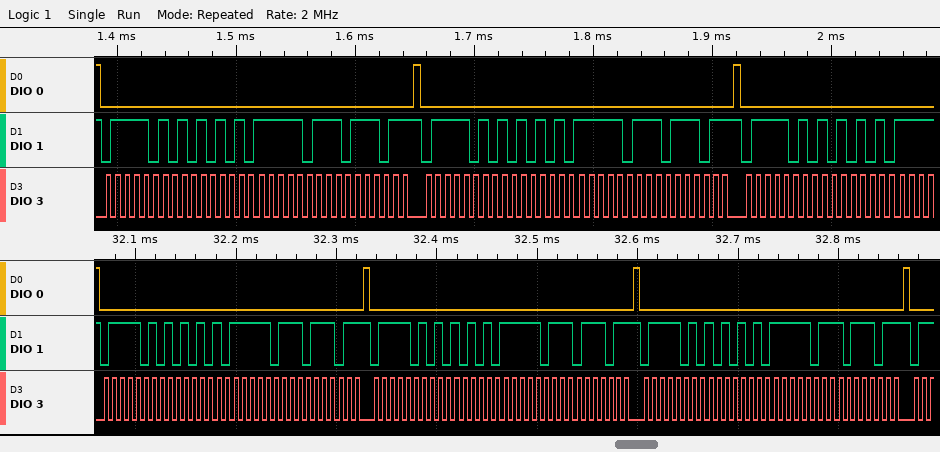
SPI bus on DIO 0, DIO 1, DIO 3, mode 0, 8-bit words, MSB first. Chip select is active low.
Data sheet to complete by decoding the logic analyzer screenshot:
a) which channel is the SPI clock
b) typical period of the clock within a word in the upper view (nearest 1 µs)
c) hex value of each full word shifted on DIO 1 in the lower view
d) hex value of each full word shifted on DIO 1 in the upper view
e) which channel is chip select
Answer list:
DIO 3
8 µs
7A, AA, FB, BB, 7A, AA, FB, BB, 7A, AA, FB, BB
7A, AA, FB, BB, 7A, AA, FB, BB, 7A, AA
DIO 0
